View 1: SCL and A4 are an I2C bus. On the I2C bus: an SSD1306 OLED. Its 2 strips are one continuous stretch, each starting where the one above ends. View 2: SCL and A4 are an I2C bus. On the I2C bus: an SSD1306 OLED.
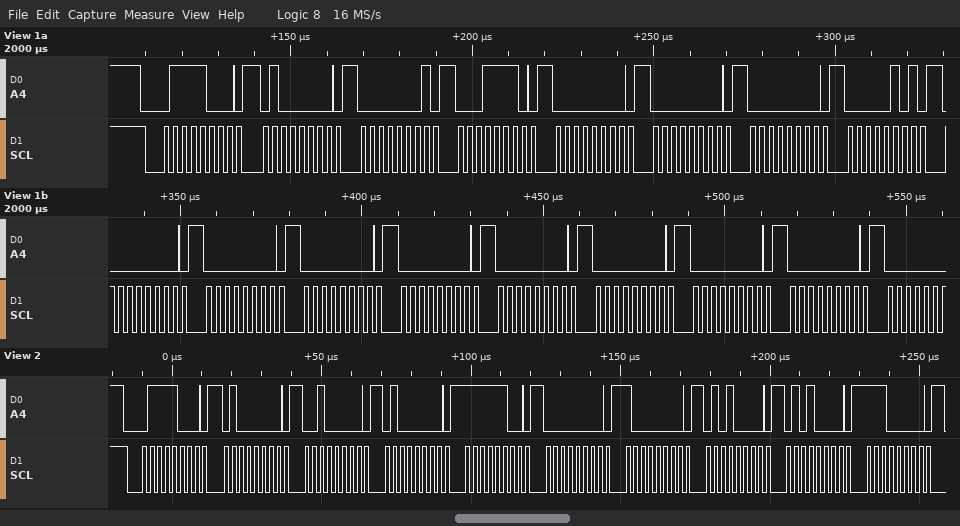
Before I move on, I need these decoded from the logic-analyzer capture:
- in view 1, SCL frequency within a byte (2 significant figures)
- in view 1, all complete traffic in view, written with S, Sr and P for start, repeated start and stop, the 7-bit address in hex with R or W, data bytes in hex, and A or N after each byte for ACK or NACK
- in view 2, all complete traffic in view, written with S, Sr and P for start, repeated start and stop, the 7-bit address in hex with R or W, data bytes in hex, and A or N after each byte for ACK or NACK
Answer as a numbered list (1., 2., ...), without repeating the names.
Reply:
1. 400 kHz
2. S 3CW A 40 A 01 A 1E A 00 A 00 A 00 A 05 A 00 A 00 A 00 A 00 A 00 A 00 A 00 A 00 A
3. S 3CW A 40 A 20 A 40 A FC A 00 A 80 A 50 A 50 A E0 A
